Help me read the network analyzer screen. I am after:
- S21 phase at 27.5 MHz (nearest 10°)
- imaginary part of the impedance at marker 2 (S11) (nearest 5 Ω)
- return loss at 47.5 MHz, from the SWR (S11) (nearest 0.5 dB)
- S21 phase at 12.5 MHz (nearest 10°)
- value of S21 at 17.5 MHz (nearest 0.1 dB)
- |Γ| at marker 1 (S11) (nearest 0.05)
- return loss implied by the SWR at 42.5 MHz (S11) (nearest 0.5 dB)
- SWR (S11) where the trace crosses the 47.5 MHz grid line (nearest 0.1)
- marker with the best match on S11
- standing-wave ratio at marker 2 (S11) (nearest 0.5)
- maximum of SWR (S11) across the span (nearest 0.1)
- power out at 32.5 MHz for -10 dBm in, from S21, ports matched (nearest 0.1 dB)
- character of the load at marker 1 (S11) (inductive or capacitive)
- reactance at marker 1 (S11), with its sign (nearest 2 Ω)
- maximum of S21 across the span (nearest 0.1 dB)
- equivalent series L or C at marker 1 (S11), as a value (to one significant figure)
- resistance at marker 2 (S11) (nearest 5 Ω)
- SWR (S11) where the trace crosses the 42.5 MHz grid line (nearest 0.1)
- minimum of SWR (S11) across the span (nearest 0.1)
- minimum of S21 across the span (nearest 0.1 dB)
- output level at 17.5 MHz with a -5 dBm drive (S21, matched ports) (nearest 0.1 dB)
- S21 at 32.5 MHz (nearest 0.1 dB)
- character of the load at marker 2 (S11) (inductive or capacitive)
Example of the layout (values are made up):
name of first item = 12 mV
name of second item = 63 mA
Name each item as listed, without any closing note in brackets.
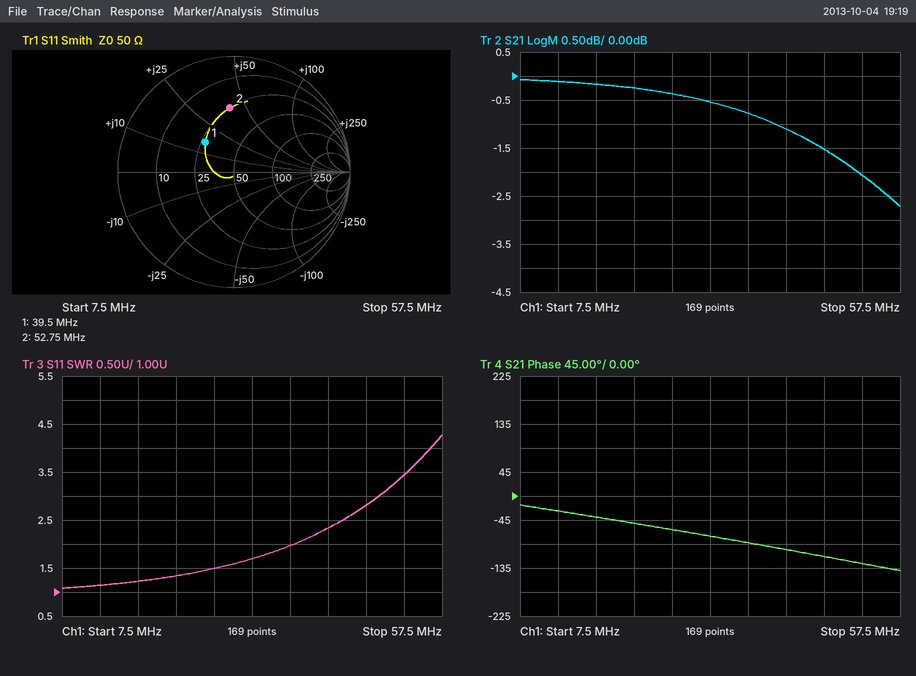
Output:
S21 phase at 27.5 MHz = -60°
imaginary part of the impedance at marker 2 (S11) = +40 Ω
return loss at 47.5 MHz, from the SWR (S11) = 6.5 dB
S21 phase at 12.5 MHz = -30°
value of S21 at 17.5 MHz = -0.2 dB
|Γ| at marker 1 (S11) = 0.35
return loss implied by the SWR at 42.5 MHz (S11) = 8.0 dB
SWR (S11) where the trace crosses the 47.5 MHz grid line = 2.8
marker with the best match on S11 = marker 1
standing-wave ratio at marker 2 (S11) = 3.5
maximum of SWR (S11) across the span = 4.3
power out at 32.5 MHz for -10 dBm in, from S21, ports matched = -10.5 dBm
character of the load at marker 1 (S11) = inductive
reactance at marker 1 (S11), with its sign = +16 Ω
maximum of S21 across the span = -0.1 dB
equivalent series L or C at marker 1 (S11), as a value = 60 nH
resistance at marker 2 (S11) = 25 Ω
SWR (S11) where the trace crosses the 42.5 MHz grid line = 2.3
minimum of SWR (S11) across the span = 1.1
minimum of S21 across the span = -2.7 dB
output level at 17.5 MHz with a -5 dBm drive (S21, matched ports) = -5.2 dBm
S21 at 32.5 MHz = -0.5 dB
character of the load at marker 2 (S11) = inductive
